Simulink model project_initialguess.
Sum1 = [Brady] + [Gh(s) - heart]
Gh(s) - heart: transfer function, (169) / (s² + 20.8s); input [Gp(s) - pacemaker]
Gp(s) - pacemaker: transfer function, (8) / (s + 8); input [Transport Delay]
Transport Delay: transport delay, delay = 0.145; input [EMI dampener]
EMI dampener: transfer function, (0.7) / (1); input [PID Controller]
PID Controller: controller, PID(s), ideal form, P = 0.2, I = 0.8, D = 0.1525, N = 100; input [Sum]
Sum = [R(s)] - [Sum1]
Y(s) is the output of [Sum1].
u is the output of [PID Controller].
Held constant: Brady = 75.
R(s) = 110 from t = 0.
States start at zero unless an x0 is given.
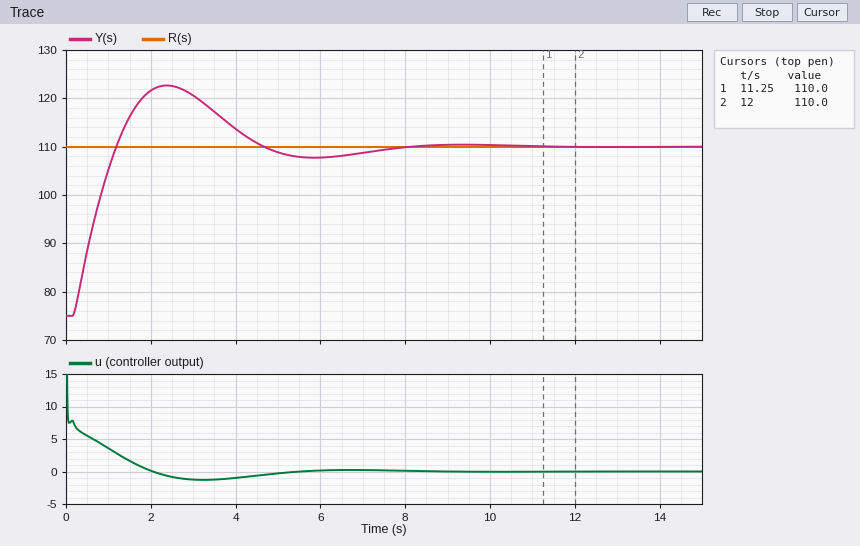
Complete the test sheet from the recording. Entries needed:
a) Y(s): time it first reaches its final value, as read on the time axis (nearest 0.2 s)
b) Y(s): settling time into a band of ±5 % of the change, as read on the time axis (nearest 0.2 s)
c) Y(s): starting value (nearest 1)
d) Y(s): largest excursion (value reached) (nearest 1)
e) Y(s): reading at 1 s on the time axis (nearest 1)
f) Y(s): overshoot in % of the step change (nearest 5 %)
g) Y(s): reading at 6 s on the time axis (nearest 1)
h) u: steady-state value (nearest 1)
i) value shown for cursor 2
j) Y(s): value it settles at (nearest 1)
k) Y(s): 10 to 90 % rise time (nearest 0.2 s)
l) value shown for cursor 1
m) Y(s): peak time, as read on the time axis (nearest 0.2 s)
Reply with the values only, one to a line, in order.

1.2 s
6.6 s
75
123
105
35 %
108
0
110.0
110
0.8 s
110.0
2.4 s
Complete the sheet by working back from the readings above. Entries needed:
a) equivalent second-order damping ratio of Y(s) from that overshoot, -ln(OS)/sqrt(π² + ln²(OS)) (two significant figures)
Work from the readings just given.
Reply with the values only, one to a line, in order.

0.32
